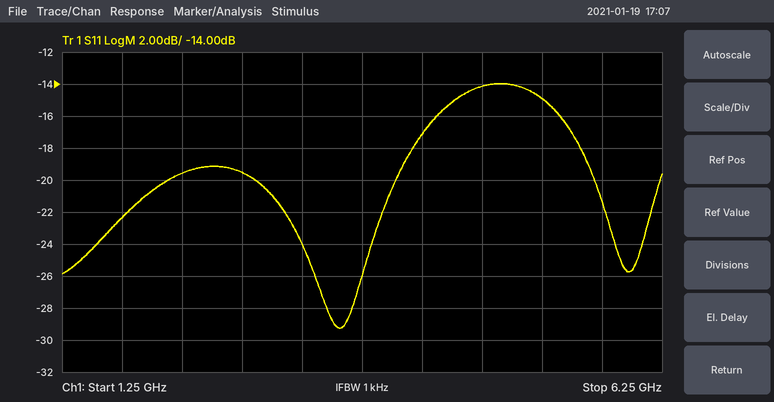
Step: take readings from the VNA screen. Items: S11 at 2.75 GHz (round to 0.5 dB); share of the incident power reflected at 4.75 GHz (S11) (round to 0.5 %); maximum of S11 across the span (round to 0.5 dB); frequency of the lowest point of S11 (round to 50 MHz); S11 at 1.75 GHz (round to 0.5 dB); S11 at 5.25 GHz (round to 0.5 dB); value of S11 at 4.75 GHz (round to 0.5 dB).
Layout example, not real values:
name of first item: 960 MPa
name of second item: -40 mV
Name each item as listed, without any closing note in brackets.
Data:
S11 at 2.75 GHz: -19.5 dB
share of the incident power reflected at 4.75 GHz (S11): 4.0 %
maximum of S11 across the span: -14.0 dB
frequency of the lowest point of S11: 3.55 GHz
S11 at 1.75 GHz: -22.5 dB
S11 at 5.25 GHz: -15.0 dB
value of S11 at 4.75 GHz: -14.0 dB
